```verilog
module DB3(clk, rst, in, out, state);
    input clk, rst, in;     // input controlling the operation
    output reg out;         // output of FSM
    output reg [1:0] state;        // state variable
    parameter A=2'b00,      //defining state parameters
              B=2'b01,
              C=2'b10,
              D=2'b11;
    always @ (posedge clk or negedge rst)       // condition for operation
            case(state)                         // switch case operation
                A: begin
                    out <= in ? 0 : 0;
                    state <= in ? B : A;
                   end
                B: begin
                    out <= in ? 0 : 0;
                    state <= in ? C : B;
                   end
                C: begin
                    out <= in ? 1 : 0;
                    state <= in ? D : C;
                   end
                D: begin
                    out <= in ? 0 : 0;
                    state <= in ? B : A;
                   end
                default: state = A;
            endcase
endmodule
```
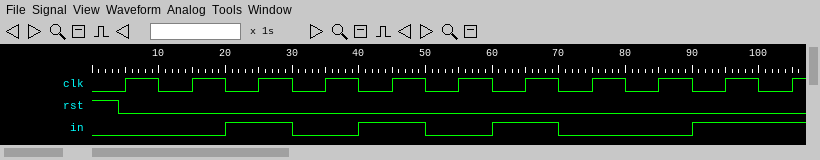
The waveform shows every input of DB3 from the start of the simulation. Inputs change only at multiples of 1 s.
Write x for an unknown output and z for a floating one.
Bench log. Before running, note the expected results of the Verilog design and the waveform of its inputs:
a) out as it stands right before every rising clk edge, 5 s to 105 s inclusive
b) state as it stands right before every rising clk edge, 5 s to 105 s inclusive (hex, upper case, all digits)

x 0 0 0 0 0 0 1 0 0 0
0, 0, 0, 1, 1, 2, 2, 3, 0, 0, 1
